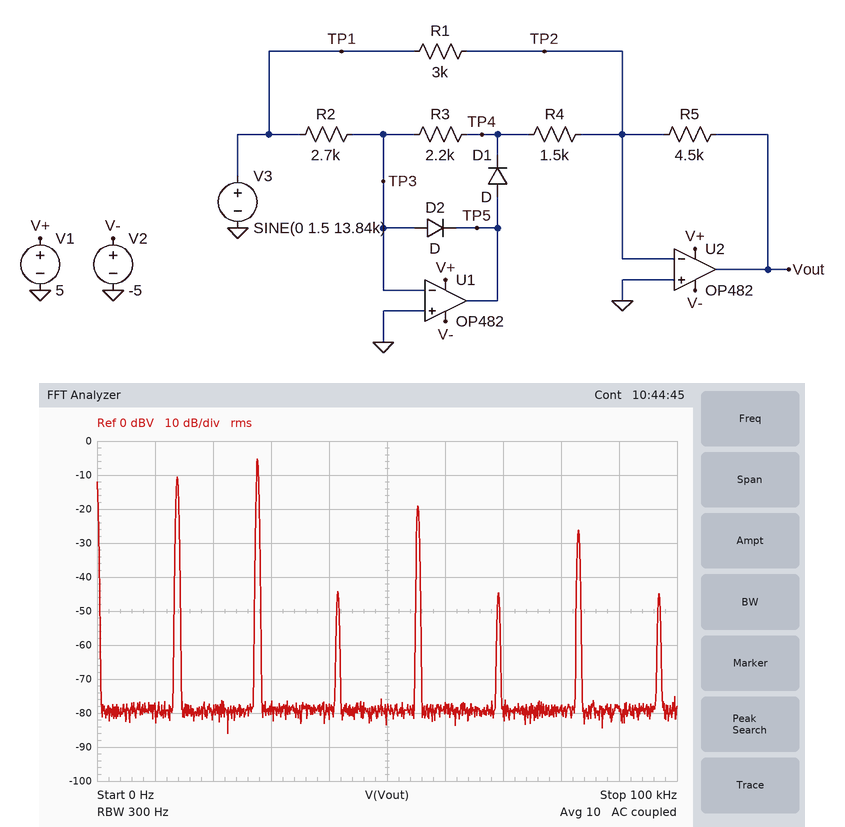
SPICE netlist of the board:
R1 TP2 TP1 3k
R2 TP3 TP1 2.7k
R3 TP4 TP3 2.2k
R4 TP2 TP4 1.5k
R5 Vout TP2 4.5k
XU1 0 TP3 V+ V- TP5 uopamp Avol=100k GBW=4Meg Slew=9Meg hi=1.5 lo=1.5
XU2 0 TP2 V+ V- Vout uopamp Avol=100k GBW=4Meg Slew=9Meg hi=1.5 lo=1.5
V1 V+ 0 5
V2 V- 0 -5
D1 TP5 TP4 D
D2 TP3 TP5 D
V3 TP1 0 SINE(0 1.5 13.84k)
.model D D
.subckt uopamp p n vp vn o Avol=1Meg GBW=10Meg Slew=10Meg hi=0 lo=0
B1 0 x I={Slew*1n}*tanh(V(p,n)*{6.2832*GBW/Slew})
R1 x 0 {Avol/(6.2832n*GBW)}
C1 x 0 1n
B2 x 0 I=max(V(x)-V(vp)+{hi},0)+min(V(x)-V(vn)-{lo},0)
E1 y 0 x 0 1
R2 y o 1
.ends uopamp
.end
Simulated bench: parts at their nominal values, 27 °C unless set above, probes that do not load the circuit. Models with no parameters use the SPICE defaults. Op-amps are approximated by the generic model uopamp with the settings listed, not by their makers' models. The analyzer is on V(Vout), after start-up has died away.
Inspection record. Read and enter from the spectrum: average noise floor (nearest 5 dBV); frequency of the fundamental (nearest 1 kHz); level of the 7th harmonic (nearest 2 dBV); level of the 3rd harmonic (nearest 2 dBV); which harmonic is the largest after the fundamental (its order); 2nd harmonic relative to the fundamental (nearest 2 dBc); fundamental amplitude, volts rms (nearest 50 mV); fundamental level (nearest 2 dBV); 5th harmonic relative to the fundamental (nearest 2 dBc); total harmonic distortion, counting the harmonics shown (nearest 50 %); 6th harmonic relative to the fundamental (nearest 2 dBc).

-80 dBV
14 kHz
-44 dBV
-44 dBV
2
6 dBc
300 mV
-10 dBV
-34 dBc
200 %
-16 dBc
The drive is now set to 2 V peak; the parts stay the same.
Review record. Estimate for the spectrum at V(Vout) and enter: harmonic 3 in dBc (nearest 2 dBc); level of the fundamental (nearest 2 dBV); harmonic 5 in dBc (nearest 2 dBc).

-36 dBc
-8 dBV
-36 dBc
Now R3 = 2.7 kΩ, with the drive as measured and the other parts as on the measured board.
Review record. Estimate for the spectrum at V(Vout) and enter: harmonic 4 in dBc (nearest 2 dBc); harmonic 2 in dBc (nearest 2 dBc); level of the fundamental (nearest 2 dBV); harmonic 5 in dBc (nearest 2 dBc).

16 dBc
30 dBc
-32 dBV
-12 dBc
